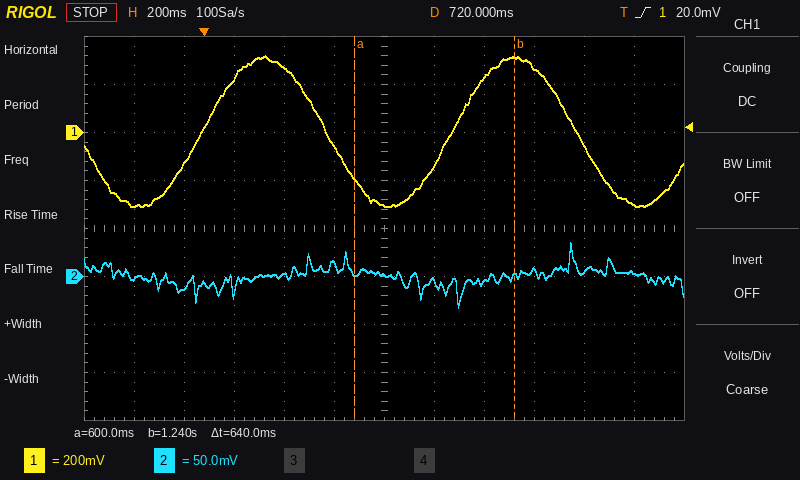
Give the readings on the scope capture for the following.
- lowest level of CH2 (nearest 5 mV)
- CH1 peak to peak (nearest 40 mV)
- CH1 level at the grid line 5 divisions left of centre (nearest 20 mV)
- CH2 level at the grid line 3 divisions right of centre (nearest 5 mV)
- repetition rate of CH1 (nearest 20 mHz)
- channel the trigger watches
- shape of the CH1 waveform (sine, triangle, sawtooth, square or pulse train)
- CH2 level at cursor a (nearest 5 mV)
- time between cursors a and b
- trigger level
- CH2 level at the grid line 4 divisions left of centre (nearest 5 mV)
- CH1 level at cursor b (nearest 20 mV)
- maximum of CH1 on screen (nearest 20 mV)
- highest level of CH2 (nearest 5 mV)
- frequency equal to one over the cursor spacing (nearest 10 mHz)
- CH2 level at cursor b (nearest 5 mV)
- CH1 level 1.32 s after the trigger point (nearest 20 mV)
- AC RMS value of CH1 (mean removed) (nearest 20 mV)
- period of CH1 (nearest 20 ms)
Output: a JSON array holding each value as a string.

["-30 mV", "640 mV", "-300 mV", "5 mV", "1.00 Hz", "CH1", "sine", "5 mV", "640 ms", "20.0 mV", "-10 mV", "320 mV", "320 mV", "35 mV", "1.56 Hz", "0 mV", "280 mV", "220 mV", "1.00 s"]
